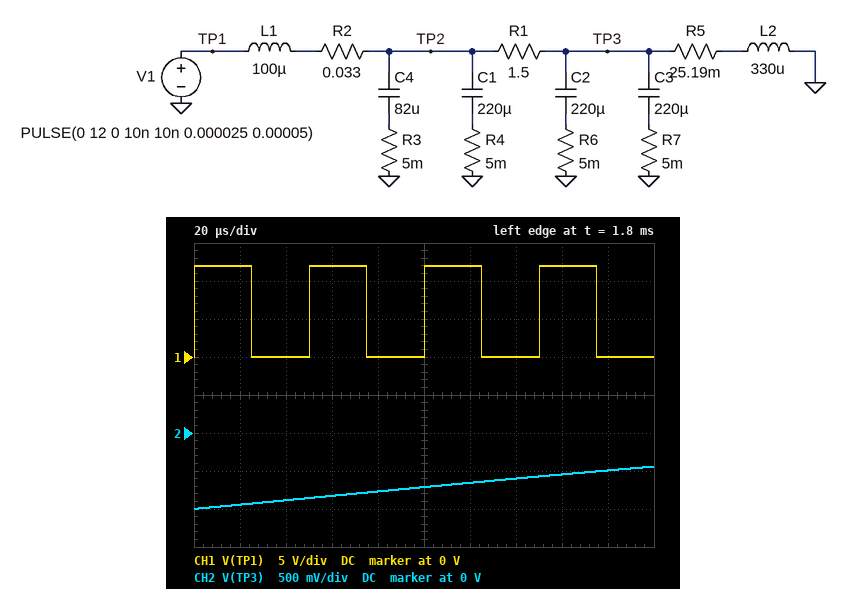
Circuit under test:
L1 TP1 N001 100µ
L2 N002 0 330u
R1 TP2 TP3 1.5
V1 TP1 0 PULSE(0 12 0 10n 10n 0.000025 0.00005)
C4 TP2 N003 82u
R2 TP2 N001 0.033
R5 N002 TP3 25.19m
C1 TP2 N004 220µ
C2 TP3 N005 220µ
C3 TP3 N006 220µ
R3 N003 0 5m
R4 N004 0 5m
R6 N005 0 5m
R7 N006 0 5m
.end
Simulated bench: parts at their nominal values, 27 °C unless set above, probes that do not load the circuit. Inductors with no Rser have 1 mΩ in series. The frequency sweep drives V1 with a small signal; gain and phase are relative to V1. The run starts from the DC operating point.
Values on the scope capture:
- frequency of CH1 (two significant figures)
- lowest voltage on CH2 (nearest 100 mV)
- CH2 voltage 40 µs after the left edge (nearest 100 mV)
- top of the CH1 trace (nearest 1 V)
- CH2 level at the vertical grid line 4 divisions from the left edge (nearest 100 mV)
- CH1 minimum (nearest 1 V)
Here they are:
20 kHz
-1.0 V
-900 mV
12 V
-800 mV
0 V
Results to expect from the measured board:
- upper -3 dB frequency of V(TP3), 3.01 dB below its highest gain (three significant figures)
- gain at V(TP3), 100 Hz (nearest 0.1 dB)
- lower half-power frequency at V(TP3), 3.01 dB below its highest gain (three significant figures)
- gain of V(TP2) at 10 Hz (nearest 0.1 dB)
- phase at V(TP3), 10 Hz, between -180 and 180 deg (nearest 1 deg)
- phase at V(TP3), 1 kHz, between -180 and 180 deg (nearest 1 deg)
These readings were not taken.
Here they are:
846 Hz
-17.0 dB
360 Hz
-0.2 dB
37 deg
165 deg
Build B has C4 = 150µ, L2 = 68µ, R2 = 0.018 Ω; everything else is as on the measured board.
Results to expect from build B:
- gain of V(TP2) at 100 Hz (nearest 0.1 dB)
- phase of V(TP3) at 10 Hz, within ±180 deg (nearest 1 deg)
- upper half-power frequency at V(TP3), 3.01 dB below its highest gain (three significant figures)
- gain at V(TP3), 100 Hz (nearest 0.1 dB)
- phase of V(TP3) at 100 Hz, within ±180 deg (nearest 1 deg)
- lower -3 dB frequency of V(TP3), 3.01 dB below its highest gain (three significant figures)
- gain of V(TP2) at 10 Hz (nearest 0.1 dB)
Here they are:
0 dB
9 deg
909 Hz
-29.6 dB
54 deg
840 Hz
-0.1 dB
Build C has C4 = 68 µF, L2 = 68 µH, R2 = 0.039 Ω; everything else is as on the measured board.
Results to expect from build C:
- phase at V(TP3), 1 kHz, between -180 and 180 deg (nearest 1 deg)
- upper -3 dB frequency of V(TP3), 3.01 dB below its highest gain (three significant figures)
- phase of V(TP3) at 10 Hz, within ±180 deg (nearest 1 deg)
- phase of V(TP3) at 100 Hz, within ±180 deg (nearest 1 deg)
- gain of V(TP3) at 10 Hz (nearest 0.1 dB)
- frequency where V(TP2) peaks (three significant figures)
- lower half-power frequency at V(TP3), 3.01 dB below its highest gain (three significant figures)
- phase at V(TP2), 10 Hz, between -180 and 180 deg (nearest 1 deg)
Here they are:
-165 deg
960 Hz
9 deg
54 deg
-35.4 dB
926 Hz
892 Hz
0 deg
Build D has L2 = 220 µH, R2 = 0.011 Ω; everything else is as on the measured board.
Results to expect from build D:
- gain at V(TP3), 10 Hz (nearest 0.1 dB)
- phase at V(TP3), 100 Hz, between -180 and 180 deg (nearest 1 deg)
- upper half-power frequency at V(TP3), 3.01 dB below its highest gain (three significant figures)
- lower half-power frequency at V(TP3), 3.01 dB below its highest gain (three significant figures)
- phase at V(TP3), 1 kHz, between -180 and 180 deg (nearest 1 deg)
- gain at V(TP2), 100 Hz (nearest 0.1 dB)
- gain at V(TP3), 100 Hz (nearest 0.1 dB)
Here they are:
-34.3 dB
71 deg
864 Hz
485 Hz
162 deg
0 dB
-20.4 dB
